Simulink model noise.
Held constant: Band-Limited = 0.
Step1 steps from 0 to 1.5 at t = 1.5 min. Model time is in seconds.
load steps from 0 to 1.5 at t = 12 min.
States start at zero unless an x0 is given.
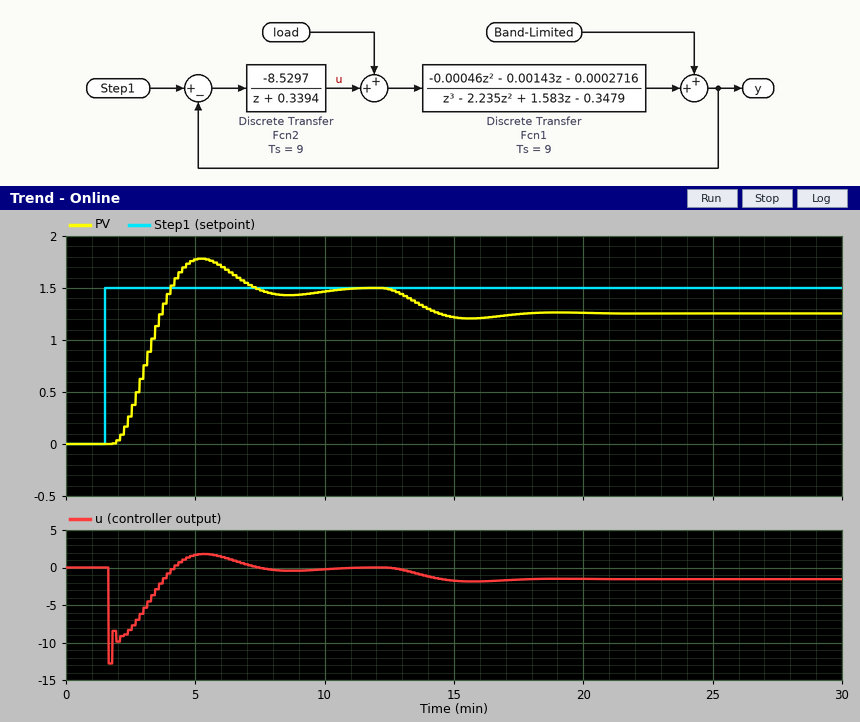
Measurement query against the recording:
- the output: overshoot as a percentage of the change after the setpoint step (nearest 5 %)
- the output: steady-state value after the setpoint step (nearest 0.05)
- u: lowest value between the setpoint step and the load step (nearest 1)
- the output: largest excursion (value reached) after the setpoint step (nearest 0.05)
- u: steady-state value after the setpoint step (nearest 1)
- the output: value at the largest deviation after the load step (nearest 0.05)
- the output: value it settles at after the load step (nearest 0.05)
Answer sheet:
20 %
1.50
-13
1.80
0
1.20
1.25
